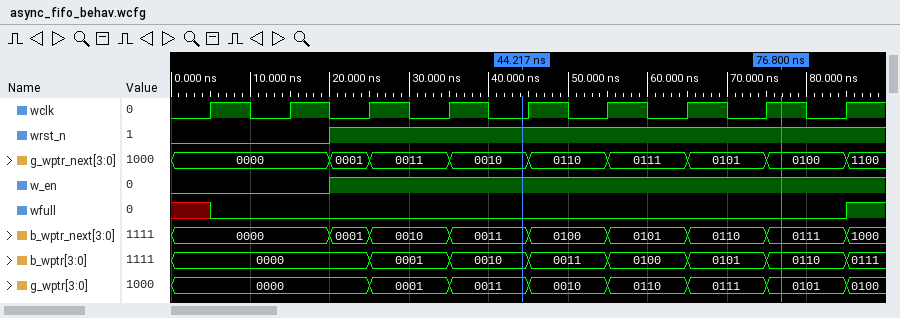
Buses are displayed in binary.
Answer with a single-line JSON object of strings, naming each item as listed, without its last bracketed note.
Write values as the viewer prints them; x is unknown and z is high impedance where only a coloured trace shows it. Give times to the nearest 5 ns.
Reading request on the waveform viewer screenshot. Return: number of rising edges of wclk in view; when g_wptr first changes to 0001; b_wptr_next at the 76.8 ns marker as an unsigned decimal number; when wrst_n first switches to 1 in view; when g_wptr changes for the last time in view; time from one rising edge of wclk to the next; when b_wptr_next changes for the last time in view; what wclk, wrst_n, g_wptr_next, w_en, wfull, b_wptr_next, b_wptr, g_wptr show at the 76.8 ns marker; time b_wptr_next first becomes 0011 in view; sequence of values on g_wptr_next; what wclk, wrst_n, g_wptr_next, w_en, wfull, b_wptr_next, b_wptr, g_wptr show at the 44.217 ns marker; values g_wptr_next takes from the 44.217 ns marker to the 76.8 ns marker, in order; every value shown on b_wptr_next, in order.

{"number of rising edges of wclk in view": "9", "when g_wptr first changes to 0001": "25 ns", "b_wptr_next at the 76.8 ns marker as an unsigned decimal number": "7", "when wrst_n first switches to 1 in view": "20 ns", "when g_wptr changes for the last time in view": "85 ns", "time from one rising edge of wclk to the next": "10 ns", "when b_wptr_next changes for the last time in view": "85 ns", "what wclk, wrst_n, g_wptr_next, w_en, wfull, b_wptr_next, b_wptr, g_wptr show at the 76.8 ns marker": "wclk=1, wrst_n=1, g_wptr_next=0100, w_en=1, wfull=0, b_wptr_next=0111, b_wptr=0110, g_wptr=0101", "time b_wptr_next first becomes 0011 in view": "35 ns", "sequence of values on g_wptr_next": "0000, 0001, 0011, 0010, 0110, 0111, 0101, 0100, 1100", "what wclk, wrst_n, g_wptr_next, w_en, wfull, b_wptr_next, b_wptr, g_wptr show at the 44.217 ns marker": "wclk=0, wrst_n=1, g_wptr_next=0010, w_en=1, wfull=0, b_wptr_next=0011, b_wptr=0010, g_wptr=0011", "values g_wptr_next takes from the 44.217 ns marker to the 76.8 ns marker, in order": "0010, 0110, 0111, 0101, 0100", "every value shown on b_wptr_next, in order": "0000, 0001, 0010, 0011, 0100, 0101, 0110, 0111, 1000"}
